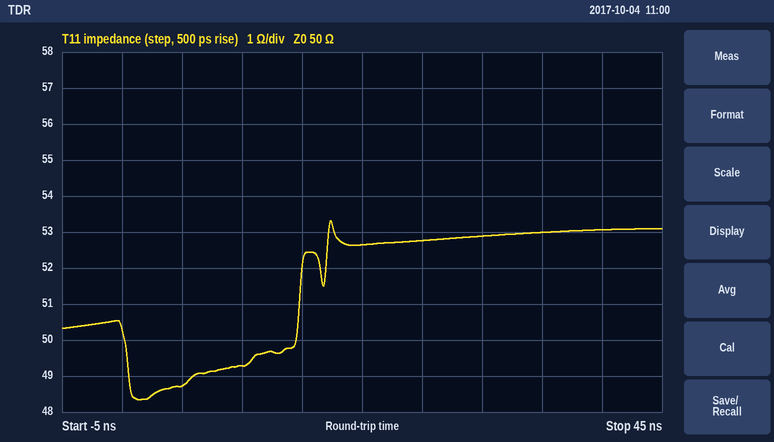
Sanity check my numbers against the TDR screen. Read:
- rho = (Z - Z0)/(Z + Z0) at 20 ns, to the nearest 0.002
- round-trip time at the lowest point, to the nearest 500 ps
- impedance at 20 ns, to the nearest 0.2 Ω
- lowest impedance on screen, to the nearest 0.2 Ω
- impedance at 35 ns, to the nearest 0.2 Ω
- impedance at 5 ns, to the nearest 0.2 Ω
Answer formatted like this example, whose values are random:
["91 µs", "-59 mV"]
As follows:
["+0.026", "1.5 ns", "52.6 Ω", "48.4 Ω", "53.0 Ω", "48.8 Ω"]
